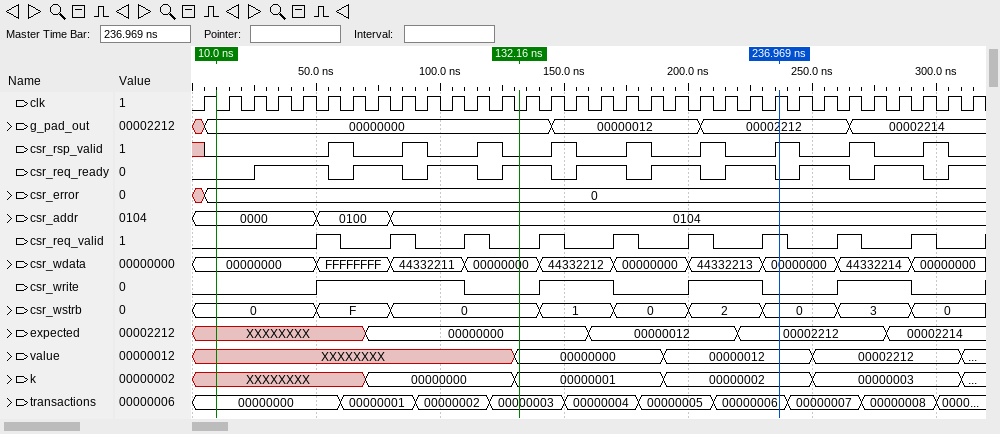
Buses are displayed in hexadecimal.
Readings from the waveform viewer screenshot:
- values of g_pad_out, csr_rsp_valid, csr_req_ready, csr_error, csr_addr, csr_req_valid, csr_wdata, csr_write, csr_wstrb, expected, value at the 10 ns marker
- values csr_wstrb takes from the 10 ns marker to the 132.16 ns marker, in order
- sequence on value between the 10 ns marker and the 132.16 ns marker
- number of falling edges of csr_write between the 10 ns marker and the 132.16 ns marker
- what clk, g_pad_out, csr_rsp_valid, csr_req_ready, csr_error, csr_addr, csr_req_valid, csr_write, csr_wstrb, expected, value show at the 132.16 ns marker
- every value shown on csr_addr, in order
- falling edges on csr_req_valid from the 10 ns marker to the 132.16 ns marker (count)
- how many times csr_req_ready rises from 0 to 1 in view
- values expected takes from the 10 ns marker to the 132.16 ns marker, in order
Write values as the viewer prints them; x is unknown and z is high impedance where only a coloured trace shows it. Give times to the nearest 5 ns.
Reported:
g_pad_out=00000000, csr_rsp_valid=0, csr_req_ready=0, csr_error=0, csr_addr=0000, csr_req_valid=0, csr_wdata=00000000, csr_write=0, csr_wstrb=0, expected=XXXXXXXX, value=XXXXXXXX
0, F, 0
XXXXXXXX, 00000000
1
clk=0, g_pad_out=00000000, csr_rsp_valid=0, csr_req_ready=1, csr_error=0, csr_addr=0104, csr_req_valid=0, csr_write=0, csr_wstrb=0, expected=00000000, value=00000000
0000, 0100, 0104
3
10
XXXXXXXX, 00000000
